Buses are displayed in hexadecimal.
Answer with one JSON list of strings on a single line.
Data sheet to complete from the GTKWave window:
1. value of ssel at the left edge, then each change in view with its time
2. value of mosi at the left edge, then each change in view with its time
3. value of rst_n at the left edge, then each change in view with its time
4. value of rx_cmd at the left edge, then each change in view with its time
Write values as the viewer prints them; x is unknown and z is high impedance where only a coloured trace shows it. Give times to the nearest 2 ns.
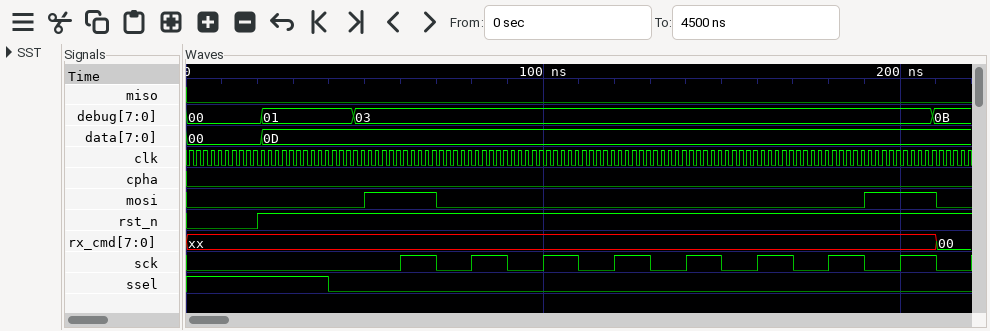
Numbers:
["1, 0 at 40 ns", "0, 1 at 50 ns, 0 at 70 ns, 1 at 190 ns, 0 at 210 ns", "0, 1 at 20 ns", "xx, 00 at 210 ns"]
